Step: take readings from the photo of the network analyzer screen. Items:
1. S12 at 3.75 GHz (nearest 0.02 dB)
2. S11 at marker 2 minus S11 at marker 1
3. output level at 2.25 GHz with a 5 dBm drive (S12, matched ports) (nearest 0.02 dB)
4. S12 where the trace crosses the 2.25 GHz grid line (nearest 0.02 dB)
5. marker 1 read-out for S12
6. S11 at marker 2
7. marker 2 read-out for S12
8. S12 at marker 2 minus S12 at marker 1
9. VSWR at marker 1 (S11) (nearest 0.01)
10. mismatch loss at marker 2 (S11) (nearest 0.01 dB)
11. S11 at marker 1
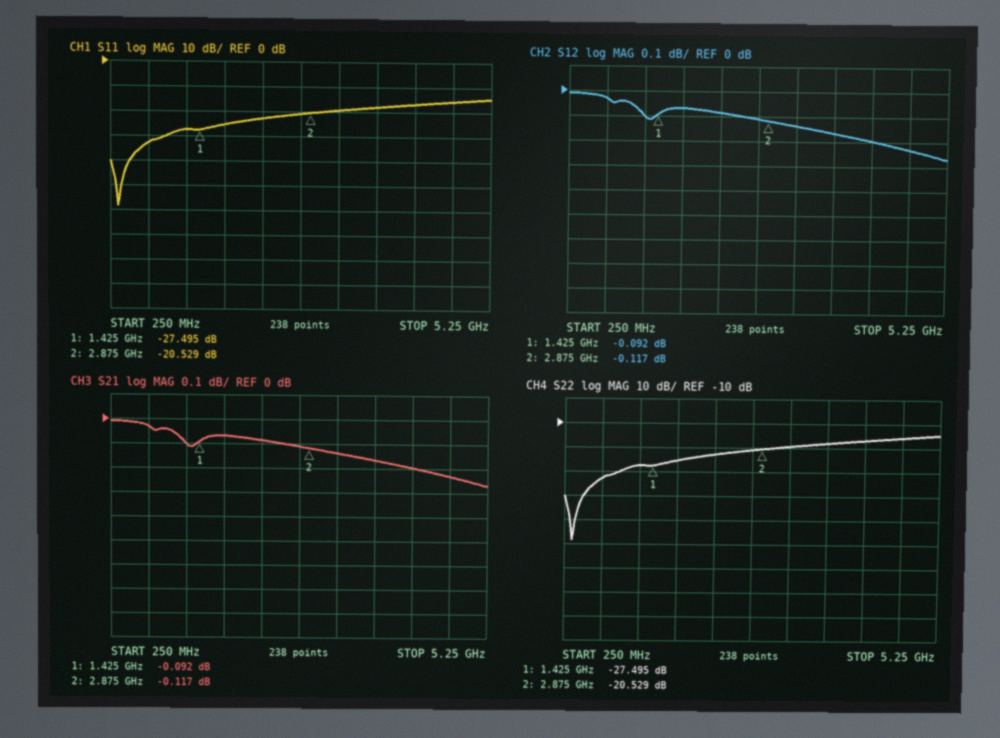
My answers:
-0.16 dB
6.966 dB
4.92 dBm
-0.08 dB
-0.092 dB
-20.529 dB
-0.117 dB
-0.025 dB
1.09
0.04 dB
-27.495 dB
